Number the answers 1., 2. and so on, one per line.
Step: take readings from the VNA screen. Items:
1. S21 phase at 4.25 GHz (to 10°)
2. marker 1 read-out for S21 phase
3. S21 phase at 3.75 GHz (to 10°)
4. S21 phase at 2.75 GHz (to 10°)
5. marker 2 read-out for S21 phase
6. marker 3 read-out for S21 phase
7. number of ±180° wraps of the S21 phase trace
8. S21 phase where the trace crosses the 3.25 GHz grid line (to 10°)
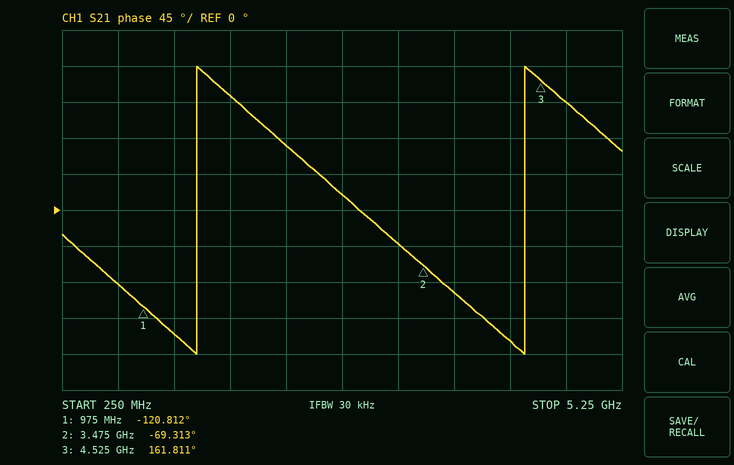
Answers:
1. -160°
2. -120.812°
3. -100°
4. 20°
5. -69.313°
6. 161.811°
7. 2
8. -40°
